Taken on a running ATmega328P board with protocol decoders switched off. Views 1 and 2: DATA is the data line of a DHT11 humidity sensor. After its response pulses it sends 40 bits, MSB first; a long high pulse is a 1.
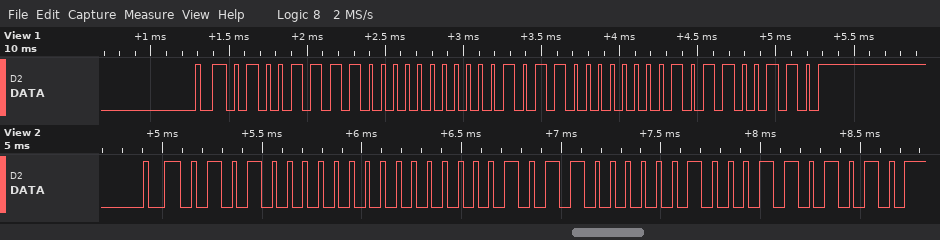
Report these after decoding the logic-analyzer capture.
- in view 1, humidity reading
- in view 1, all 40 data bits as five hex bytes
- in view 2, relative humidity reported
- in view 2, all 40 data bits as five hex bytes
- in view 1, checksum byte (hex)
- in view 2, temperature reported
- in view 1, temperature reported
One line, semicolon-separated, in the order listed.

79 %; 4F 00 16 01 66; 80 %; 50 00 16 04 6A; 0x66; 22.4 °C; 22.1 °C
